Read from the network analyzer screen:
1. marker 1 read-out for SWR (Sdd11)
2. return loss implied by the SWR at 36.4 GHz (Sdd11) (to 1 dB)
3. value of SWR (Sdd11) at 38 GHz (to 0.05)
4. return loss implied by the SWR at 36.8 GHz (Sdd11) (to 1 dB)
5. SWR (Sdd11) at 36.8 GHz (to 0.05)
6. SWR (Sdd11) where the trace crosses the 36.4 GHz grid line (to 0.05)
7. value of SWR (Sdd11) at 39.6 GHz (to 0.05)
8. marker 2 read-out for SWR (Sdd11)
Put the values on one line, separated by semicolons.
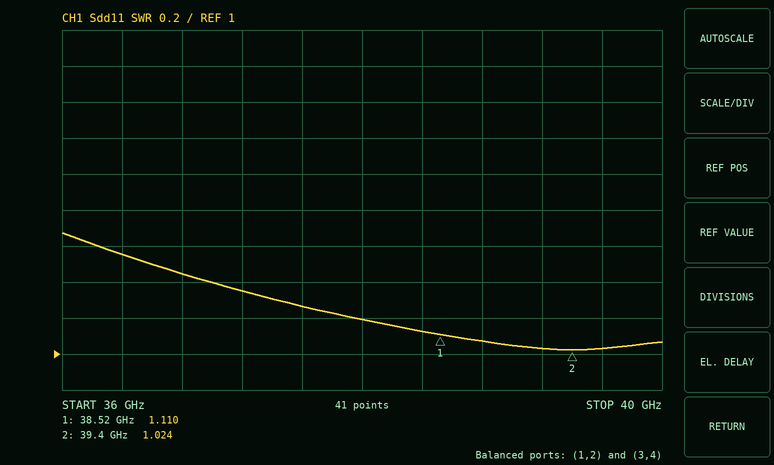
1.110; 13 dB; 1.20; 15 dB; 1.45; 1.55; 1.05; 1.024
